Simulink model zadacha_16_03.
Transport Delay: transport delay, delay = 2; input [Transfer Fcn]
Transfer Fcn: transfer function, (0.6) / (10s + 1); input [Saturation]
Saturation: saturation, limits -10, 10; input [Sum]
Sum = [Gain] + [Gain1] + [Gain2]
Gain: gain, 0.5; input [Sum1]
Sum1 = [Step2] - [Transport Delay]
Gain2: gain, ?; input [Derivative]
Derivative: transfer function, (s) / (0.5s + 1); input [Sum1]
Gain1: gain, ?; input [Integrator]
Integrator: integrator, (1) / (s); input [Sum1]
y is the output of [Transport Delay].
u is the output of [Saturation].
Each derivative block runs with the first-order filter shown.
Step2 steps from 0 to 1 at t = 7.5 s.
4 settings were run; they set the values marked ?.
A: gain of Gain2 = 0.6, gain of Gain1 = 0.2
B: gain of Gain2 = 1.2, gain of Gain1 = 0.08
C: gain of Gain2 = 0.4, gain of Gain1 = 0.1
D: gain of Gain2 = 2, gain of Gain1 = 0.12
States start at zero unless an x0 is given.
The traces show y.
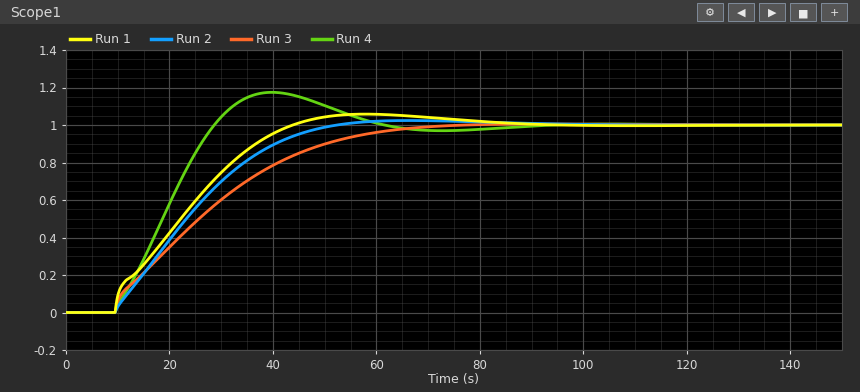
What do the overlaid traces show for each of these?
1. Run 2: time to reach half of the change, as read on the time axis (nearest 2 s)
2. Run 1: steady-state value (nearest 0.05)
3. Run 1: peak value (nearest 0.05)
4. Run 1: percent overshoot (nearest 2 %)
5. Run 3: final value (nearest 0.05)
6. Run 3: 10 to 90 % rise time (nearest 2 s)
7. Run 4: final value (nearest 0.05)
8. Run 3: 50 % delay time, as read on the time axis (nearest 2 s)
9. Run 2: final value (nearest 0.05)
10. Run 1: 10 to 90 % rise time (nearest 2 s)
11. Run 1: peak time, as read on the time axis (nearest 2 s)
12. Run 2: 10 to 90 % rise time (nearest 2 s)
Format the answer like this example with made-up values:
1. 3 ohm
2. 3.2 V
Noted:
1. 24 s
2. 1.00
3. 1.05
4. 6 %
5. 1.00
6. 40 s
7. 1.00
8. 26 s
9. 1.00
10. 26 s
11. 58 s
12. 28 s
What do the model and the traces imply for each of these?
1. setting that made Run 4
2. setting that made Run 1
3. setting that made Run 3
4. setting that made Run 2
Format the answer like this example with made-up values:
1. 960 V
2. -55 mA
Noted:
1. A
2. D
3. B
4. C
